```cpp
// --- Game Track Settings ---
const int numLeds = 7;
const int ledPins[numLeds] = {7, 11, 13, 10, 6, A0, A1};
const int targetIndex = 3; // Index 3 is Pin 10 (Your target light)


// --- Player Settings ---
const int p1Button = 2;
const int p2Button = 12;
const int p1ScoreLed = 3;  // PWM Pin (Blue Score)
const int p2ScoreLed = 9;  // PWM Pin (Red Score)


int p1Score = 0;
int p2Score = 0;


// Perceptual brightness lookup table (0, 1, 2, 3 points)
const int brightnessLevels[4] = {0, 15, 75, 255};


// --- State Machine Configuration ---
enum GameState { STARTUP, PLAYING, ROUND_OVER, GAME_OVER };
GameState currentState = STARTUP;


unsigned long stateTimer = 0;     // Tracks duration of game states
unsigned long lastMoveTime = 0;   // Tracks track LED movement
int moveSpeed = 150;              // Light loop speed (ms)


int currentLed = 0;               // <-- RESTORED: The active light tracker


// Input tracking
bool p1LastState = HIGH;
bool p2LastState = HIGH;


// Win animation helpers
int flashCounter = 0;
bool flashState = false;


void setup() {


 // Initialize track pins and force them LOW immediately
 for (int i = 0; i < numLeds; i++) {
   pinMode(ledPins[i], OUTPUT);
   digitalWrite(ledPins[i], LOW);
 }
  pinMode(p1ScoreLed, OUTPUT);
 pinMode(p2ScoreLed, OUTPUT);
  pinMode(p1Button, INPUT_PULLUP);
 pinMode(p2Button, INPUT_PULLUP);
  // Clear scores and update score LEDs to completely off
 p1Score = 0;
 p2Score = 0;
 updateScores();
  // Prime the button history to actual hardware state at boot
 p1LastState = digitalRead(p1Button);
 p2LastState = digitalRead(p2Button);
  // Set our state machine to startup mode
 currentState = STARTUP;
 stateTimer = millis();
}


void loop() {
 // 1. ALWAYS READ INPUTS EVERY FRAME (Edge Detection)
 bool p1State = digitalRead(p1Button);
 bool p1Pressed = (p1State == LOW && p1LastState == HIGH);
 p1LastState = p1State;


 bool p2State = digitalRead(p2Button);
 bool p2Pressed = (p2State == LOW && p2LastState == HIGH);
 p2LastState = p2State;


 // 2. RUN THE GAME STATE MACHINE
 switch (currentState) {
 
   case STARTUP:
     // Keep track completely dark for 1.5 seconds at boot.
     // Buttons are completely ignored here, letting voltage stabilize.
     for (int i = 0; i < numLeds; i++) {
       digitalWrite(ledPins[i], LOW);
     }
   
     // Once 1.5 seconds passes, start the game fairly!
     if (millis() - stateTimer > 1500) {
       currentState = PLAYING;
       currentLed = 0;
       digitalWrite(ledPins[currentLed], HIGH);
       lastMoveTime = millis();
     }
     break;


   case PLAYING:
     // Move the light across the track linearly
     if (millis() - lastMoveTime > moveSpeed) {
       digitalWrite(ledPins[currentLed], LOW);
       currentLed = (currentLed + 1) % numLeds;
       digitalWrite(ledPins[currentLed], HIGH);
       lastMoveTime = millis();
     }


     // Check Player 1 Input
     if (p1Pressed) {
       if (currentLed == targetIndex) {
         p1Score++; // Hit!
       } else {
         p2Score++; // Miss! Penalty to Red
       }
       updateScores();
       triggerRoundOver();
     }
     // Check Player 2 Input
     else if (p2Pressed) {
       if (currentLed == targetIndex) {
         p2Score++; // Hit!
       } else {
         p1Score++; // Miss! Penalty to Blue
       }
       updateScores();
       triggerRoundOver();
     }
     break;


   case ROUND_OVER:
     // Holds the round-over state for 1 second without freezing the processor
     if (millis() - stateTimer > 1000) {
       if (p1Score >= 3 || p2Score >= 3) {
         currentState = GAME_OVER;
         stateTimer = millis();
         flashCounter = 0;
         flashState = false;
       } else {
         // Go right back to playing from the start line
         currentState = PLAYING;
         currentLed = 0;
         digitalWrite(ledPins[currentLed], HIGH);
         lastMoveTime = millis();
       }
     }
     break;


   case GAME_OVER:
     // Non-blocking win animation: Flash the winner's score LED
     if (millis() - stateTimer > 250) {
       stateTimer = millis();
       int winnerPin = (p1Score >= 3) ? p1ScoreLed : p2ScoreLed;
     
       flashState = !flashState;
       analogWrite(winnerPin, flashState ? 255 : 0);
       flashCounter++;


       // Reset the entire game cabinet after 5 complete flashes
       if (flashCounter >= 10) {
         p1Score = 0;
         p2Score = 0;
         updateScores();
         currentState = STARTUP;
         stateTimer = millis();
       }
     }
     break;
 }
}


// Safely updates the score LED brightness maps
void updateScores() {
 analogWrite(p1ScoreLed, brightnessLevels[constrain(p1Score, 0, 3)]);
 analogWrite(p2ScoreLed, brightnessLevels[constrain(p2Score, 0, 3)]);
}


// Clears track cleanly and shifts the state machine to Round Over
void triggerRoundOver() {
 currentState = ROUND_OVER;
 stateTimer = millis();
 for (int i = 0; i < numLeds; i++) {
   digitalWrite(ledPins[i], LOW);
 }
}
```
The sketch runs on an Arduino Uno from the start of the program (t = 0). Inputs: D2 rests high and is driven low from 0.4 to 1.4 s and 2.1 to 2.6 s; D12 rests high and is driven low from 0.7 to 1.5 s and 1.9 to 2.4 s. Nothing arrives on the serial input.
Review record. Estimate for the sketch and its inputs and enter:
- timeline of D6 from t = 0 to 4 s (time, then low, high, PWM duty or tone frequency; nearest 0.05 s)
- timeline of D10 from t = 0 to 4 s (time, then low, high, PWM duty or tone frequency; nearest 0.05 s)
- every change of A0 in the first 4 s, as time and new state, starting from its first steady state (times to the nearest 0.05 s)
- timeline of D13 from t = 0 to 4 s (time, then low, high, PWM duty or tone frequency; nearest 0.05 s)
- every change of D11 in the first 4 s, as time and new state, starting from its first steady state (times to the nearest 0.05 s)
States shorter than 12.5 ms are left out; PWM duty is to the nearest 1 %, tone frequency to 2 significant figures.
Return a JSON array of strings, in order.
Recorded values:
["0 s low; 3.5 s high; 3.65 s low", "0 s low; 3.35 s high; 3.5 s low", "0 s low; 3.65 s high; 3.8 s low", "0 s low; 1.8 s high; 1.9 s low; 3.2 s high; 3.35 s low", "0 s low; 1.65 s high; 1.8 s low; 3.05 s high; 3.2 s low"]
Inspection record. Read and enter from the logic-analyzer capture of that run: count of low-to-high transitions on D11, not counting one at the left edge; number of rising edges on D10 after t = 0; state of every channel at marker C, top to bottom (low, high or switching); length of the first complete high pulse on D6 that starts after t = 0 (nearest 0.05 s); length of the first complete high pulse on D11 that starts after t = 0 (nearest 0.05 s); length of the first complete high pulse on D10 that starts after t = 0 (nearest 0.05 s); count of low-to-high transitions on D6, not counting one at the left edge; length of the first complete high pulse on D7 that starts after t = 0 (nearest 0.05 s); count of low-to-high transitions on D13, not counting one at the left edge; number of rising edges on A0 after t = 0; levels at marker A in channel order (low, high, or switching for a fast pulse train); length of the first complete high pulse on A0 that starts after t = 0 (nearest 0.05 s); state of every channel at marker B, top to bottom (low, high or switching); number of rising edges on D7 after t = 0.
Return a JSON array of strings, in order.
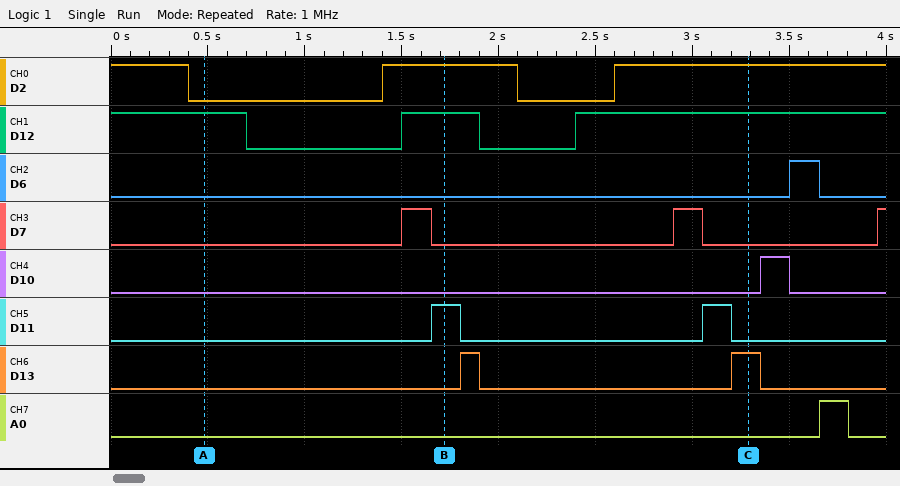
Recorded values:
["2", "1", "D2 high, D12 high, D6 low, D7 low, D10 low, D11 low, D13 high, A0 low", "0.15 s", "0.15 s", "0.15 s", "1", "0.15 s", "2", "1", "D2 low, D12 high, D6 low, D7 low, D10 low, D11 low, D13 low, A0 low", "0.15 s", "D2 high, D12 high, D6 low, D7 low, D10 low, D11 high, D13 low, A0 low", "3"]
